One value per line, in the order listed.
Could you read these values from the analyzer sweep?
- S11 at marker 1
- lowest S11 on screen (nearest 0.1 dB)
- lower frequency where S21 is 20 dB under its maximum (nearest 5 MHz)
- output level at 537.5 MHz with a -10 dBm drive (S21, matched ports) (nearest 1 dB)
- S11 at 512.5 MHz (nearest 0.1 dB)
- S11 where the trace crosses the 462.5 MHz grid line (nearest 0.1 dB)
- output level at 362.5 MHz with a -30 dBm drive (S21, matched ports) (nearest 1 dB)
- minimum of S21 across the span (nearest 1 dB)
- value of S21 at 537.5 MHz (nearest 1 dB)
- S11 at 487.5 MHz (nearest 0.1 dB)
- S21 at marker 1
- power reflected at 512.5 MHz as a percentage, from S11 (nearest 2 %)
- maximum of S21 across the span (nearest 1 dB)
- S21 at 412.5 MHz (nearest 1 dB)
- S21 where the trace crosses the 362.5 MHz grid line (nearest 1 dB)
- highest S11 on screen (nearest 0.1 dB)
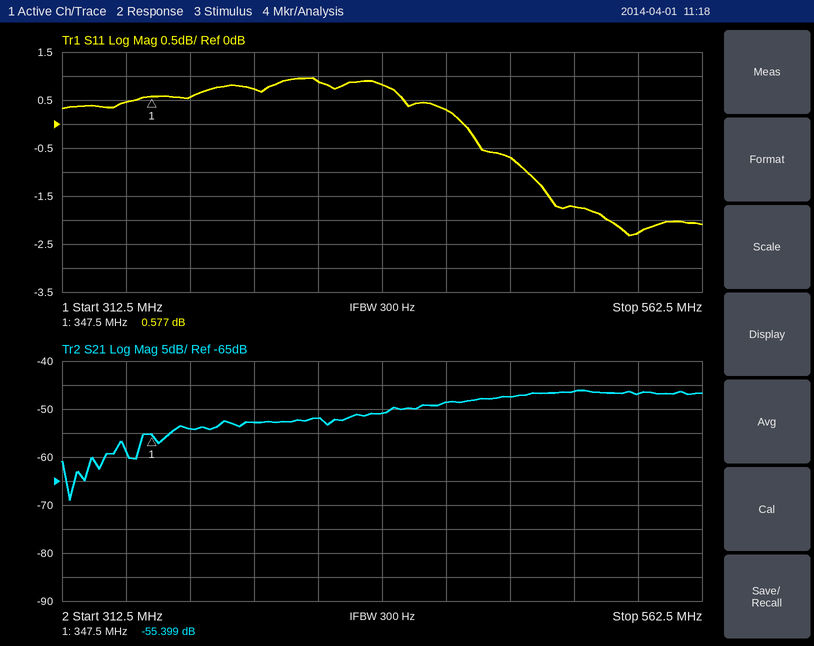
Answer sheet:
0.577 dB
-2.3 dB
315 MHz
-57 dBm
-1.7 dB
0.3 dB
-84 dBm
-69 dB
-47 dB
-0.7 dB
-55.399 dB
68 %
-46 dB
-52 dB
-54 dB
1.0 dB
